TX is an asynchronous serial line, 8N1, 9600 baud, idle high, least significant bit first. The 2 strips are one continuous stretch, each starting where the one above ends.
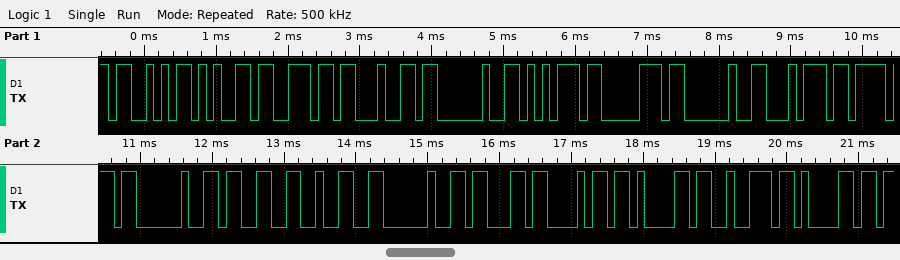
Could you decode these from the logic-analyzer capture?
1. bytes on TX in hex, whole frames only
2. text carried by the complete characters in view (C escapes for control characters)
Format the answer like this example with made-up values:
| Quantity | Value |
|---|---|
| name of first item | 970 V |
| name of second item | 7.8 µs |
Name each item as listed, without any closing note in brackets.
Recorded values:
| Quantity | Value |
|---|---|
| bytes on TX in hex, whole frames only | 53 65 6E 64 20 75 70 20 74 6F 20 33 32 20 63 68 61 72 61 |
| text carried by the complete characters in view | "Send up to 32 chara" |
